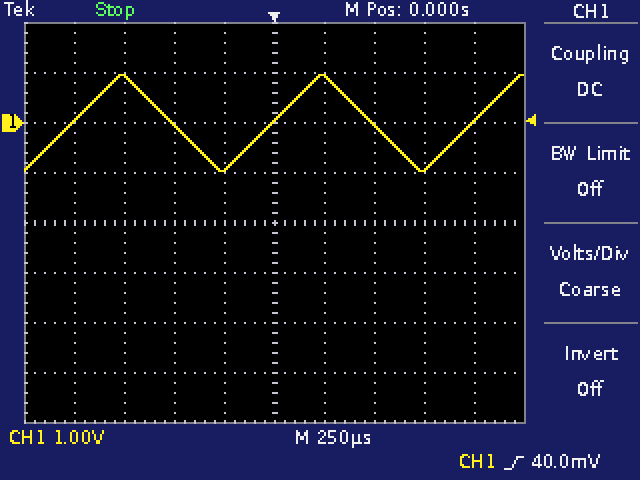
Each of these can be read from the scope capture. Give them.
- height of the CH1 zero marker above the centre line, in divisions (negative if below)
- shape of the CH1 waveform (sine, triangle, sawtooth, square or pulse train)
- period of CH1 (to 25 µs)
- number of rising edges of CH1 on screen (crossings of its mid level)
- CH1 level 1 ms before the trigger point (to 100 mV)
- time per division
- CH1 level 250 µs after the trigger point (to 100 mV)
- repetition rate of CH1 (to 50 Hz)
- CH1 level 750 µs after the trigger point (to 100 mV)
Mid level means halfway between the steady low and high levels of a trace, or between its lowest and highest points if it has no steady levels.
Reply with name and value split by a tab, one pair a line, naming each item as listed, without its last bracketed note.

height of the CH1 zero marker above the centre line, in divisions	+2.0 div
shape of the CH1 waveform	triangle
period of CH1	1.000 ms
number of rising edges of CH1 on screen	3
CH1 level 1 ms before the trigger point	0.0 V
time per division	250 µs
CH1 level 250 µs after the trigger point	900 mV
repetition rate of CH1	1.00 kHz
CH1 level 750 µs after the trigger point	-900 mV
